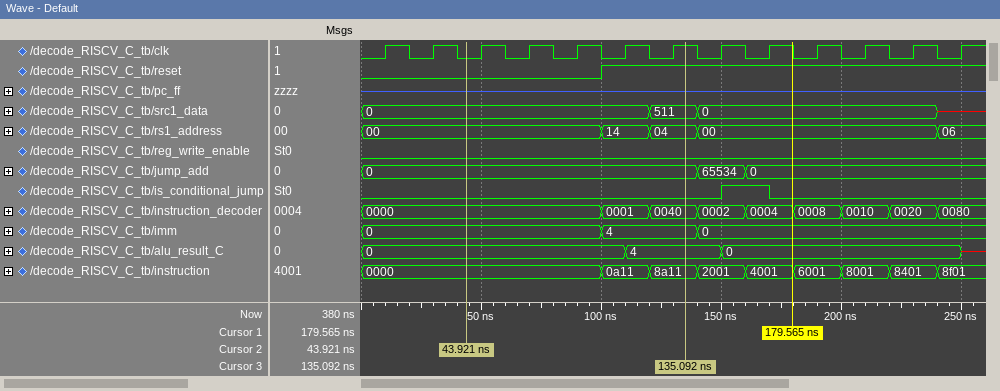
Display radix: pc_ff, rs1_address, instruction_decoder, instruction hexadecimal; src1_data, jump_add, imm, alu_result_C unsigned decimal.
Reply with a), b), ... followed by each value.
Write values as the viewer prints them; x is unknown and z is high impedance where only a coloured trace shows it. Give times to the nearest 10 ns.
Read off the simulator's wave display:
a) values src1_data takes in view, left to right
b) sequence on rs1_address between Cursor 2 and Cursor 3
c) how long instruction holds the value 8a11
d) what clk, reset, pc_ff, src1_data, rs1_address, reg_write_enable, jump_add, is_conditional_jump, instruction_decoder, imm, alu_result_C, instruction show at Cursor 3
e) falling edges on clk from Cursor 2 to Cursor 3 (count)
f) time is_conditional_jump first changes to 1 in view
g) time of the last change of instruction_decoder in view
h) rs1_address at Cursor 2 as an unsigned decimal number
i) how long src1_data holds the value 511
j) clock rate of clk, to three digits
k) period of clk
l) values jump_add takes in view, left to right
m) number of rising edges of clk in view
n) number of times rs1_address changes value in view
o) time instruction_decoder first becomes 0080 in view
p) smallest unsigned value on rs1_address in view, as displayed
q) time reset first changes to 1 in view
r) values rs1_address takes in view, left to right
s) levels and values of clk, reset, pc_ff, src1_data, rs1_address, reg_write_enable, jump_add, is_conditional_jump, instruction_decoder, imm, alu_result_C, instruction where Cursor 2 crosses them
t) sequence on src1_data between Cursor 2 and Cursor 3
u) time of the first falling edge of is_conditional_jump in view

a) 0, 511, 0, x
b) 00, 14, 04
c) 20 ns
d) clk=1, reset=1, pc_ff=z, src1_data=511, rs1_address=04, reg_write_enable=0, jump_add=0, is_conditional_jump=0, instruction_decoder=0040, imm=4, alu_result_C=4, instruction=8a11
e) 4
f) 150 ns
g) 240 ns
h) 0
i) 20 ns
j) 50.0 MHz
k) 20 ns
l) 0, 65534, 0
m) 13
n) 4
o) 240 ns
p) 00
q) 100 ns
r) 00, 14, 04, 00, 06
s) clk=0, reset=0, pc_ff=z, src1_data=0, rs1_address=00, reg_write_enable=0, jump_add=0, is_conditional_jump=0, instruction_decoder=0000, imm=0, alu_result_C=0, instruction=0000
t) 0, 511
u) 170 ns
